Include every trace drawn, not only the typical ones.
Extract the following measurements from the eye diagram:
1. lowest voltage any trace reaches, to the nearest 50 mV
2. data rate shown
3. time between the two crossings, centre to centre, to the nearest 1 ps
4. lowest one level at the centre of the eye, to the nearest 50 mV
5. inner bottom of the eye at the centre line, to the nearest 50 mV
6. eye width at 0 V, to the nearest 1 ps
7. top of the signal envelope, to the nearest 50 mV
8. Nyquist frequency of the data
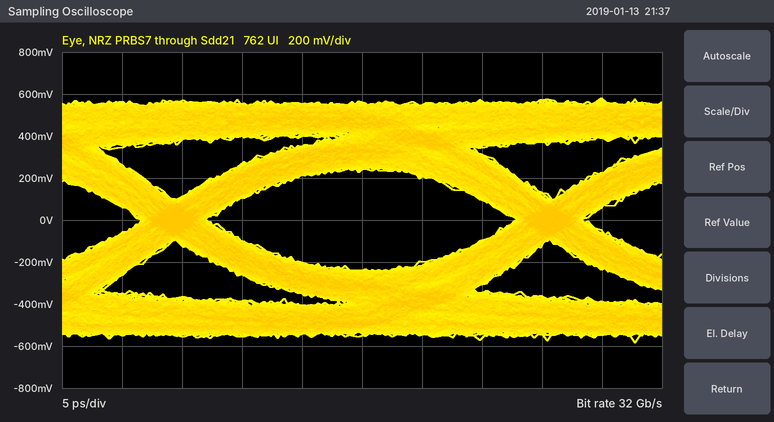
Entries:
-600 mV
32 Gb/s
31 ps
250 mV
-250 mV
26 ps
600 mV
16 GHz
